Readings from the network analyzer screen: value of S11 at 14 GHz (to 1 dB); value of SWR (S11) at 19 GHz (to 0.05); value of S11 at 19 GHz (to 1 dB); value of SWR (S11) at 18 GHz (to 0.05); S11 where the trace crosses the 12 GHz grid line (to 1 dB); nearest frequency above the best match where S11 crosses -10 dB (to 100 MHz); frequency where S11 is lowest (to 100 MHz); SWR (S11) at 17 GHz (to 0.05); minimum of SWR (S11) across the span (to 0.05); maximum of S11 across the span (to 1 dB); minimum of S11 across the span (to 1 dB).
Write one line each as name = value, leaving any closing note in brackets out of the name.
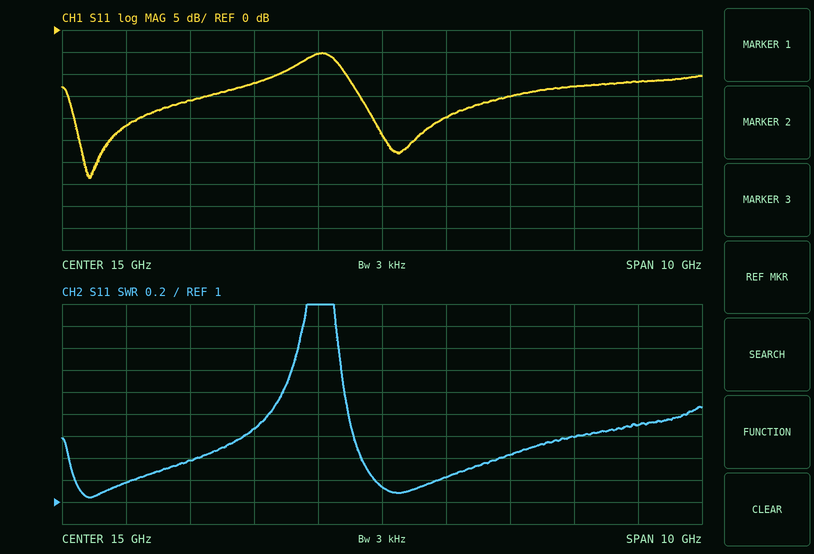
value of S11 at 14 GHz = -5 dB
value of SWR (S11) at 19 GHz = 1.70
value of S11 at 19 GHz = -12 dB
value of SWR (S11) at 18 GHz = 1.60
S11 where the trace crosses the 12 GHz grid line = -16 dB
nearest frequency above the best match where S11 crosses -10 dB = 13.4 GHz
frequency where S11 is lowest = 10.4 GHz
SWR (S11) at 17 GHz = 1.45
minimum of SWR (S11) across the span = 1.05
maximum of S11 across the span = -5 dB
minimum of S11 across the span = -34 dB
